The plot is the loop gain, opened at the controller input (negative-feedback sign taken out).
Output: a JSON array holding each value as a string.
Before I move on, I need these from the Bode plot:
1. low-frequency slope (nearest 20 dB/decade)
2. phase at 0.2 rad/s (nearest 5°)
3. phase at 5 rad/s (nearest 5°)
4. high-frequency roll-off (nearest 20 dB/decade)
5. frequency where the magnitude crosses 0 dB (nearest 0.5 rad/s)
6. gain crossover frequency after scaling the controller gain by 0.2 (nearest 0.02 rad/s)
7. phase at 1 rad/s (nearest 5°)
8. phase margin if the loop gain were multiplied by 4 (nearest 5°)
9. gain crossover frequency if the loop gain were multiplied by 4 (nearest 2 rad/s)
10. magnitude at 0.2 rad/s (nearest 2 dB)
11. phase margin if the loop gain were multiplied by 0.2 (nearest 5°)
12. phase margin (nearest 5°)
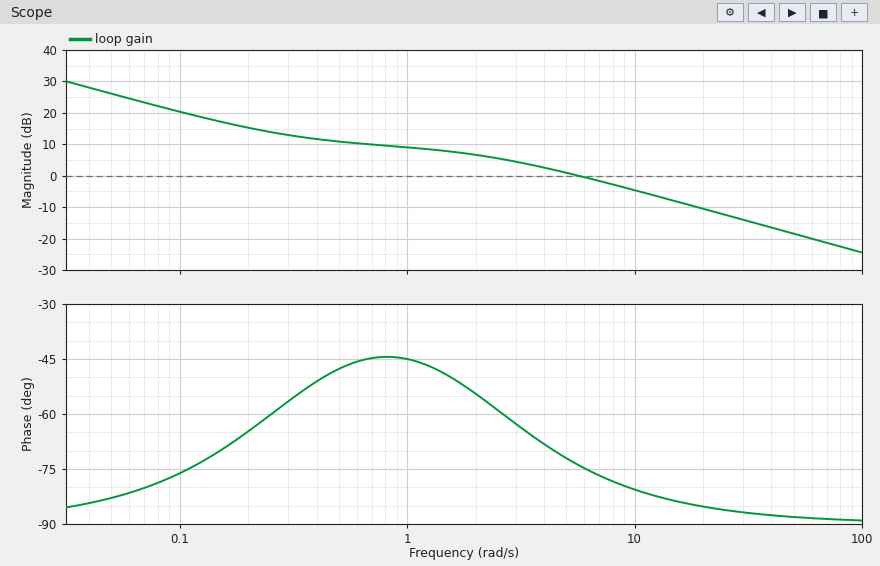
["-20 dB/decade", "-65°", "-70°", "-20 dB/decade", "5.5 rad/s", "0.24 rad/s", "-45°", "95°", "24 rad/s", "16 dB", "120°", "105°"]
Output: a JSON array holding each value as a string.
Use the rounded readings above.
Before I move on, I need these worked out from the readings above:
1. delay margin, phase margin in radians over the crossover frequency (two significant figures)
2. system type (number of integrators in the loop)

["0.33 s", "1"]
